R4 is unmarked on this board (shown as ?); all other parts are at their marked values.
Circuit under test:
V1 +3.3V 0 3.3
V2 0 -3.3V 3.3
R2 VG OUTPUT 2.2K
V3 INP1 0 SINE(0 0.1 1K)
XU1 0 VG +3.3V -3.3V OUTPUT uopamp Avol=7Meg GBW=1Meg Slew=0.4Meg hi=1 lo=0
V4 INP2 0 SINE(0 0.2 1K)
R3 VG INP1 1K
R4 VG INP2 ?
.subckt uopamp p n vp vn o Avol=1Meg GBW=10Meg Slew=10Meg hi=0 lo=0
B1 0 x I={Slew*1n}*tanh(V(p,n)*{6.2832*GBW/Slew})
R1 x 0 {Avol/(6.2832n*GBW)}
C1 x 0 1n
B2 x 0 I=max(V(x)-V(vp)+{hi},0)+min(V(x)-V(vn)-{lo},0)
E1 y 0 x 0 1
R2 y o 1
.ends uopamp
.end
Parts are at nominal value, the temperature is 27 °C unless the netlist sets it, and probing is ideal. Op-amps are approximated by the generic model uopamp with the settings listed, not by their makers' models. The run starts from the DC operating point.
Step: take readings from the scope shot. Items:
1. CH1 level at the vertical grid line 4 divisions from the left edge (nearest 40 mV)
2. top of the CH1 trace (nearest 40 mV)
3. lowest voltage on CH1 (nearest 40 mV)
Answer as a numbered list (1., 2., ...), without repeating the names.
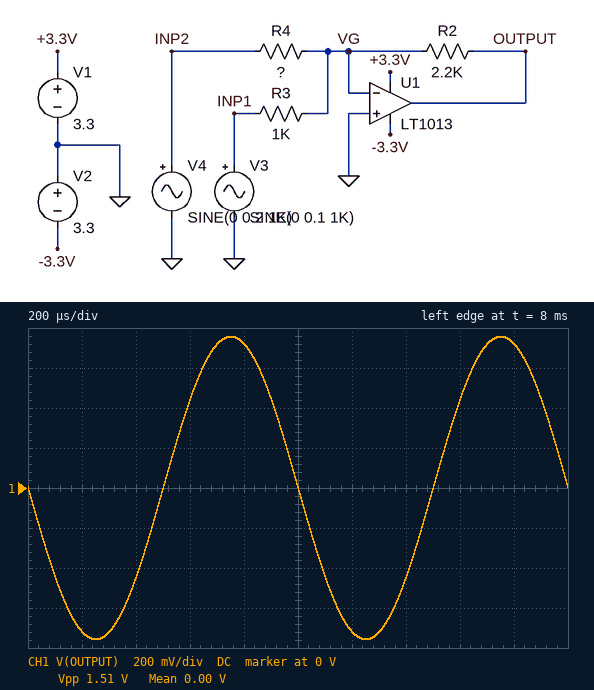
1. 720 mV
2. 760 mV
3. -760 mV
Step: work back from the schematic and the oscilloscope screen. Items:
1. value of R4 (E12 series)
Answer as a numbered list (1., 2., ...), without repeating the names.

1. 820 Ω
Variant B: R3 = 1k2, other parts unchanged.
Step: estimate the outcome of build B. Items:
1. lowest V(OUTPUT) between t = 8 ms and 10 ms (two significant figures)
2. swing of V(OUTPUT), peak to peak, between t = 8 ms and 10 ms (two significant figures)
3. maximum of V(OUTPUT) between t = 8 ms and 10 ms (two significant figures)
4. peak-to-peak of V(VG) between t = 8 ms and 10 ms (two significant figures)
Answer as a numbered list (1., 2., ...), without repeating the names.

1. -720 mV
2. 1.4 V
3. 720 mV
4. 1.4 mV
